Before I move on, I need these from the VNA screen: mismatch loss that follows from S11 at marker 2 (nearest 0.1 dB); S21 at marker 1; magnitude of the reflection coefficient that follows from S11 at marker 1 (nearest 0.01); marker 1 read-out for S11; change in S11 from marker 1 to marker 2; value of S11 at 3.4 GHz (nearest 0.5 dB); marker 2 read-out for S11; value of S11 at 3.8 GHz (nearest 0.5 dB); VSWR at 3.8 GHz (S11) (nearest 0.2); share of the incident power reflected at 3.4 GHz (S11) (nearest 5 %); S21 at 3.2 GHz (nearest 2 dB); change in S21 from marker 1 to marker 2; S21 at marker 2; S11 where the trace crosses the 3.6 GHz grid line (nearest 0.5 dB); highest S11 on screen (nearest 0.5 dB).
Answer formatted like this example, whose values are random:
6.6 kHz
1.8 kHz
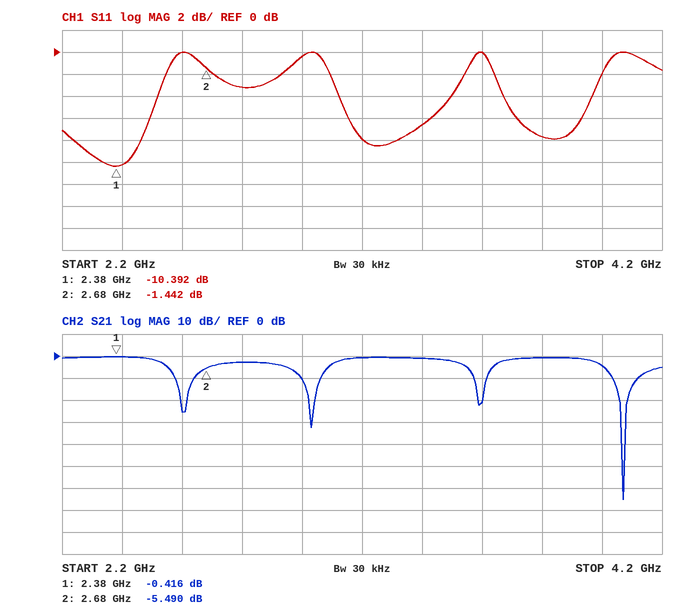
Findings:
5.5 dB
-0.416 dB
0.30
-10.392 dB
8.950 dB
-6.5 dB
-1.442 dB
-7.5 dB
2.4
20 %
0 dB
-5.074 dB
-5.490 dB
0.0 dB
0.0 dB
